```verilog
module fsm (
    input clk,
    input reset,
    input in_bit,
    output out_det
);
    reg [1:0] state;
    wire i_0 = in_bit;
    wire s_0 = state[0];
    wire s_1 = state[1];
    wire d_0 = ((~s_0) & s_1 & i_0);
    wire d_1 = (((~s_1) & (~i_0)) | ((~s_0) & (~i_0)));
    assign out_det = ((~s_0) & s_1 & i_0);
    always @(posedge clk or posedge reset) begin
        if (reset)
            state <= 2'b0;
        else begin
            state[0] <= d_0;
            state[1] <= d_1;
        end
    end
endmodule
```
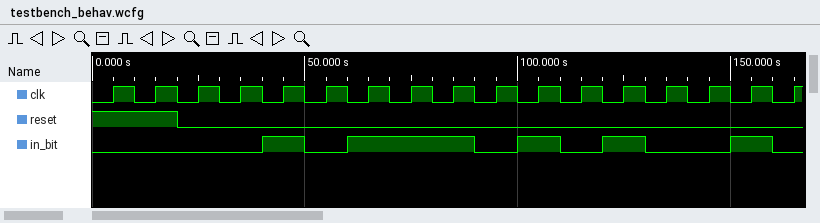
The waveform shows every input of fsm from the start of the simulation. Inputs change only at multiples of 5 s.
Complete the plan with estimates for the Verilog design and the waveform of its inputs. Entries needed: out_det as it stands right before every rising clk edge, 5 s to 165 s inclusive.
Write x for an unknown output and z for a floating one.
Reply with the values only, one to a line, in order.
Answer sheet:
0 0 0 0 1 0 1 0 0 0 1 0 1 0 0 1 0
